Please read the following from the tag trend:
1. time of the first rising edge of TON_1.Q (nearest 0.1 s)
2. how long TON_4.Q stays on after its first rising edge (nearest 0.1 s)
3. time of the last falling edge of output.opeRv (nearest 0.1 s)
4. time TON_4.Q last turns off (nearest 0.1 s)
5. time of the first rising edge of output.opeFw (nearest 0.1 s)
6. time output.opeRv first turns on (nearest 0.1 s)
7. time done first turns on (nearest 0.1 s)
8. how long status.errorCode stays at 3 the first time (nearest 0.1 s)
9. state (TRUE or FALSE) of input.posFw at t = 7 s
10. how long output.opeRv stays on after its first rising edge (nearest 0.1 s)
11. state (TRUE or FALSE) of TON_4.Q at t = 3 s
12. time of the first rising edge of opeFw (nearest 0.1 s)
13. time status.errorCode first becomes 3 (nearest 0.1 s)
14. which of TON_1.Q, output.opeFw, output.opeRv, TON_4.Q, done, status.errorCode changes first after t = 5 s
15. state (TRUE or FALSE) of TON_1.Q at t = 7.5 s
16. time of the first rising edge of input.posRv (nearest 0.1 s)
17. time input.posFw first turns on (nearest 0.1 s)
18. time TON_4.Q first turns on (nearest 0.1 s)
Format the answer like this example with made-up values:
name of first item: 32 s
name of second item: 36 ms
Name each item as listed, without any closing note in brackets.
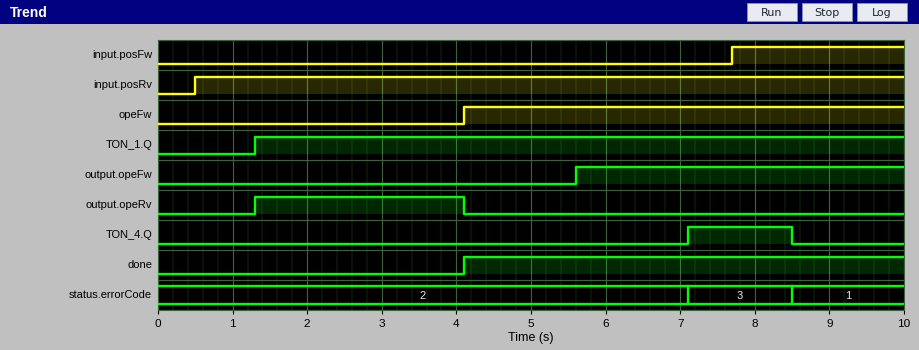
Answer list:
time of the first rising edge of TON_1.Q: 1.3 s
how long TON_4.Q stays on after its first rising edge: 1.4 s
time of the last falling edge of output.opeRv: 4.1 s
time TON_4.Q last turns off: 8.5 s
time of the first rising edge of output.opeFw: 5.6 s
time output.opeRv first turns on: 1.3 s
time done first turns on: 4.1 s
how long status.errorCode stays at 3 the first time: 1.4 s
state (TRUE or FALSE) of input.posFw at t = 7 s: FALSE
how long output.opeRv stays on after its first rising edge: 2.8 s
state (TRUE or FALSE) of TON_4.Q at t = 3 s: FALSE
time of the first rising edge of opeFw: 4.1 s
time status.errorCode first becomes 3: 7.1 s
which of TON_1.Q, output.opeFw, output.opeRv, TON_4.Q, done, status.errorCode changes first after t = 5 s: output.opeFw
state (TRUE or FALSE) of TON_1.Q at t = 7.5 s: TRUE
time of the first rising edge of input.posRv: 0.5 s
time input.posFw first turns on: 7.7 s
time TON_4.Q first turns on: 7.1 s
